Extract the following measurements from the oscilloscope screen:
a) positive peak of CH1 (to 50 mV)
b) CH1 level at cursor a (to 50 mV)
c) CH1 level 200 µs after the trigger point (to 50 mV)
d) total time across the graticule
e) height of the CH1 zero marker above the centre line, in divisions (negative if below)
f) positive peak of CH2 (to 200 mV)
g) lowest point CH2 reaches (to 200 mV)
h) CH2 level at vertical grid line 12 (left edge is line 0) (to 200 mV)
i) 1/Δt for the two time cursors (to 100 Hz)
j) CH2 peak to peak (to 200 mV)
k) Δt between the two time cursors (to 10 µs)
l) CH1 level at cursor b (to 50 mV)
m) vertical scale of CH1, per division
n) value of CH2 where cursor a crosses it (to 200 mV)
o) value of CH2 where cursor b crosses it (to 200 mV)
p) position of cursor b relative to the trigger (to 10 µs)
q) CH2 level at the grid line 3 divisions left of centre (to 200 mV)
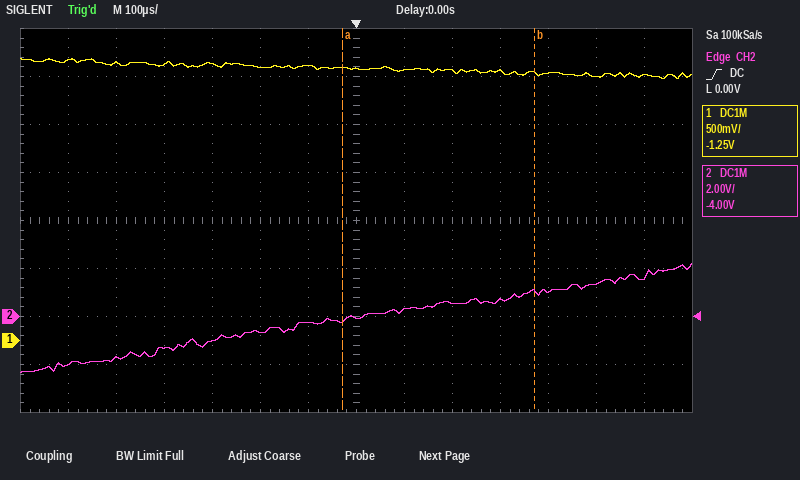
2.95 V
2.85 V
2.80 V
1.4 ms
-2.5 div
2.2 V
-2.4 V
1.4 V
2.5 kHz
4.6 V
400 µs
2.80 V
500 mV
-200 mV
1.0 V
+370 µs
-1.0 V
